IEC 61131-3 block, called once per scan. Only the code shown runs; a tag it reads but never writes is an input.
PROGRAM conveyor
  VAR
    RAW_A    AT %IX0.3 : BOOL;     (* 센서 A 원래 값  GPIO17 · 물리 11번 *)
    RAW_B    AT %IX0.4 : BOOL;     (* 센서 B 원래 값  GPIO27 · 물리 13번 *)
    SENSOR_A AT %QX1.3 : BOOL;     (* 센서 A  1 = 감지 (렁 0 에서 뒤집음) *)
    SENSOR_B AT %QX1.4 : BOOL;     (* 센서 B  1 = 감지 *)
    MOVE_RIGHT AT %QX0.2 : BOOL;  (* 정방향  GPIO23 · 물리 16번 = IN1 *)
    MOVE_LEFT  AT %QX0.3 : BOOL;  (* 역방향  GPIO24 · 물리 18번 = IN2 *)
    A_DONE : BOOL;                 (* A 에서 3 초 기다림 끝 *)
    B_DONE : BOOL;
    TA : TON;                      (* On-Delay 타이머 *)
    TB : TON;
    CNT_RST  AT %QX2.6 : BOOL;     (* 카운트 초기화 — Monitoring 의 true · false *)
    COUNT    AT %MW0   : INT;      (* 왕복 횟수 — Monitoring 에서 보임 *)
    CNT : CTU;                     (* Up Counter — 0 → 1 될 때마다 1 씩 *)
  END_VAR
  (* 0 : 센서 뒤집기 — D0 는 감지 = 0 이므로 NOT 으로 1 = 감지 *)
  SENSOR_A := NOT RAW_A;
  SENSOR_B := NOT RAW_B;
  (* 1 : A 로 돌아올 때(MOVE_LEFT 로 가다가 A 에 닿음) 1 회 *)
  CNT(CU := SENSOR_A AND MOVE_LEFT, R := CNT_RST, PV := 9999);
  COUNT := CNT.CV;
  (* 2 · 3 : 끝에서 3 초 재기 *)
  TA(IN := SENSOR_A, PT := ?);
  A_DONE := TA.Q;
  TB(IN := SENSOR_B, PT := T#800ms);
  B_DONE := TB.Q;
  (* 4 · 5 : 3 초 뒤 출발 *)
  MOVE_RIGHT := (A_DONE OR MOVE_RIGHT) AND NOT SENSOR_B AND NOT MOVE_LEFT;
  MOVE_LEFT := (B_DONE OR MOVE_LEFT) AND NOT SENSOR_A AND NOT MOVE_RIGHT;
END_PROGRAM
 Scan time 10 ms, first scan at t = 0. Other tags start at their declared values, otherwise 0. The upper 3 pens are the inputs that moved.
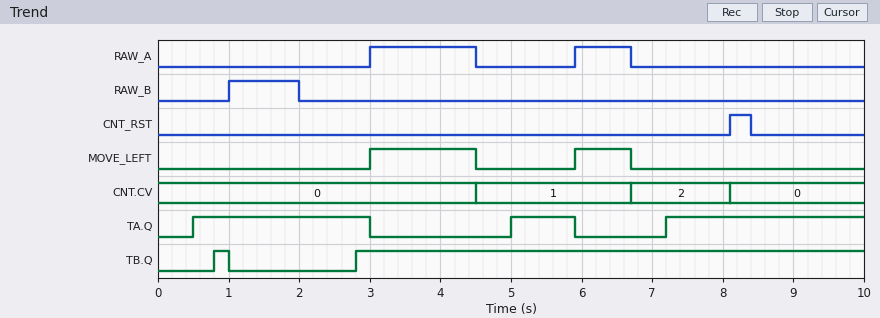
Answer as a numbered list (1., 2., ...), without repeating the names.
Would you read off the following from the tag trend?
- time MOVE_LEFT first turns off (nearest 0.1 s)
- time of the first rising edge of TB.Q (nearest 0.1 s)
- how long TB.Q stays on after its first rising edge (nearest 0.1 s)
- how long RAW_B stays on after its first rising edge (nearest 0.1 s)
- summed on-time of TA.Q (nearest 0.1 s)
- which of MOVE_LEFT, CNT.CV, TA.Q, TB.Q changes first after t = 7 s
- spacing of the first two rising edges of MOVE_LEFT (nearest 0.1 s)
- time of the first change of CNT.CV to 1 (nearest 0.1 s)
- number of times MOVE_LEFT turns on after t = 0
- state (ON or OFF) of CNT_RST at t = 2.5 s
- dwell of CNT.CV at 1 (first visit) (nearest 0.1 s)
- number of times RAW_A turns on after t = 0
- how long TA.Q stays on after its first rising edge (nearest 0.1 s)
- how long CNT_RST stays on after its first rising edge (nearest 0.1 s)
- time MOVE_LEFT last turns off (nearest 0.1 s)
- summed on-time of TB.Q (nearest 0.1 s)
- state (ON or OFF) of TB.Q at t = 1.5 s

1. 4.5 s
2. 0.8 s
3. 0.2 s
4. 1.0 s
5. 6.2 s
6. TA.Q
7. 2.9 s
8. 4.5 s
9. 2
10. OFF
11. 2.2 s
12. 2
13. 2.5 s
14. 0.3 s
15. 6.7 s
16. 7.4 s
17. OFF
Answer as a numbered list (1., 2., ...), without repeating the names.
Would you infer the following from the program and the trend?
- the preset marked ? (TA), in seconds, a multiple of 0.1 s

1. 0.5 s
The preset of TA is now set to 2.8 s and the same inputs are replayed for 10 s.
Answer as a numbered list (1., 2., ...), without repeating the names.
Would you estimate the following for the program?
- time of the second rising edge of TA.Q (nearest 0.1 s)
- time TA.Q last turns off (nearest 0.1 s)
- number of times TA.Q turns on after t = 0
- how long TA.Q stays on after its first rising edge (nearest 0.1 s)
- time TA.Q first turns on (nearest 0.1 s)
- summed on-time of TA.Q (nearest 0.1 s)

1. 9.5 s
2. 3.0 s
3. 2
4. 0.2 s
5. 2.8 s
6. 0.7 s
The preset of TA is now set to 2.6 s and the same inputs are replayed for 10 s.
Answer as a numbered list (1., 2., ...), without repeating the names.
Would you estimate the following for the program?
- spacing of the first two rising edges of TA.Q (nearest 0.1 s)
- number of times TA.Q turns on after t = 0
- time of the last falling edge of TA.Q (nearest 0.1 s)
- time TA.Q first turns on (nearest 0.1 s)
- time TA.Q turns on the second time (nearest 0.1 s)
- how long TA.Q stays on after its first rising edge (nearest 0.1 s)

1. 6.7 s
2. 2
3. 3.0 s
4. 2.6 s
5. 9.3 s
6. 0.4 s
